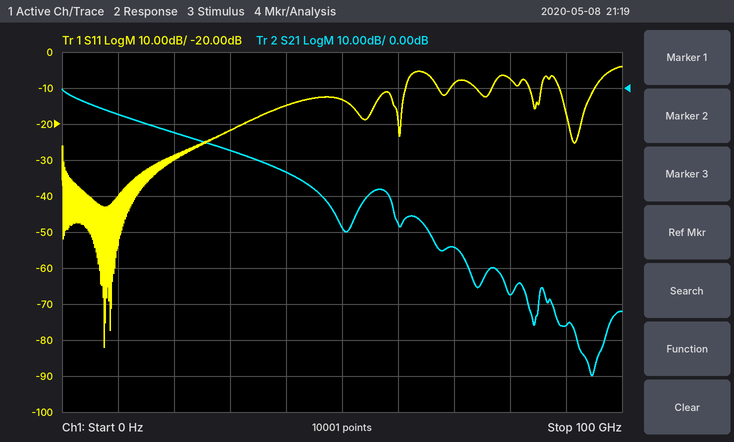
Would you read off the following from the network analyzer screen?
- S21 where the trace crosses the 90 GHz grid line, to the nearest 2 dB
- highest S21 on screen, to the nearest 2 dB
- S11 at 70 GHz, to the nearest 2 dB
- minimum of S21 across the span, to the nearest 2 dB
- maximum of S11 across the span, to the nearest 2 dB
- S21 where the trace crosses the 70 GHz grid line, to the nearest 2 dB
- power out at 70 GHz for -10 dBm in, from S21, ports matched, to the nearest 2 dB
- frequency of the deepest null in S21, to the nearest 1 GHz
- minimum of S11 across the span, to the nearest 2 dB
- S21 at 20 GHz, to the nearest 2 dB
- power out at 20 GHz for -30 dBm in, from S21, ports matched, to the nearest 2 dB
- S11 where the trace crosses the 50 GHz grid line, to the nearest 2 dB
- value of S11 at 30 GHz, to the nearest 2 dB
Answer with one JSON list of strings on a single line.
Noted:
["-66 dB", "0 dB", "-8 dB", "-80 dB", "-4 dB", "-44 dB", "-54 dBm", "95 GHz", "-82 dB", "-12 dB", "-42 dBm", "-14 dB", "-22 dB"]
